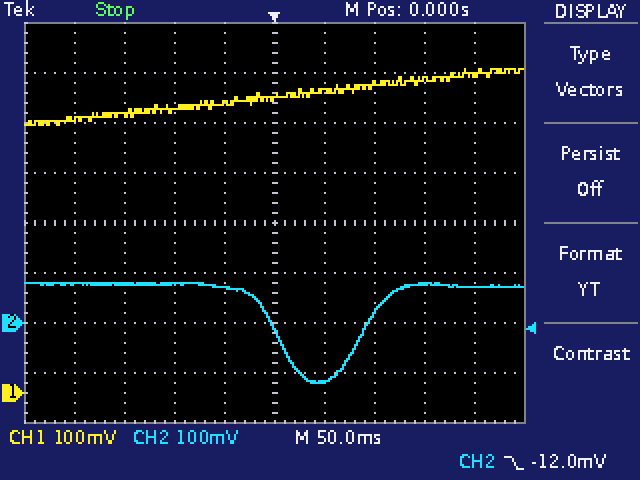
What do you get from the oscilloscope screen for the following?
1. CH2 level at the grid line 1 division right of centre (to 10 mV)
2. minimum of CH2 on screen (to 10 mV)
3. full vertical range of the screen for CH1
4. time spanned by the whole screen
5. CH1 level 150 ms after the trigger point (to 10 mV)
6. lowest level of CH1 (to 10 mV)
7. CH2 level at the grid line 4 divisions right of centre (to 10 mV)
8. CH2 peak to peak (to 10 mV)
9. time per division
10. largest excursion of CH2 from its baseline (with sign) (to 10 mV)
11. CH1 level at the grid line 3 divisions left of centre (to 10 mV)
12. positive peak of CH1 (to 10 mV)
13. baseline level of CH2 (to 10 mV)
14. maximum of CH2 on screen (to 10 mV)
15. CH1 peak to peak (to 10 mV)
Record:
-120 mV
-120 mV
800 mV
500 ms
630 mV
540 mV
70 mV
200 mV
50 ms
-200 mV
560 mV
650 mV
80 mV
80 mV
110 mV
